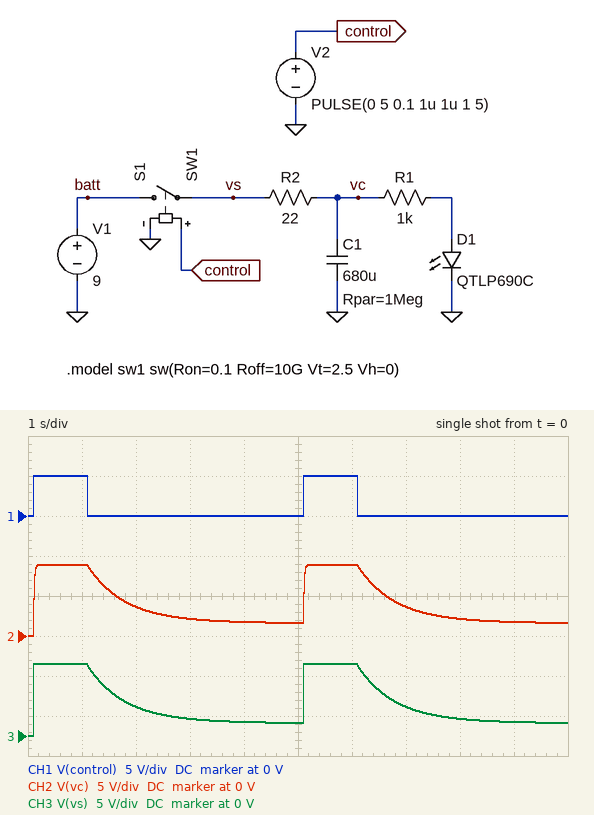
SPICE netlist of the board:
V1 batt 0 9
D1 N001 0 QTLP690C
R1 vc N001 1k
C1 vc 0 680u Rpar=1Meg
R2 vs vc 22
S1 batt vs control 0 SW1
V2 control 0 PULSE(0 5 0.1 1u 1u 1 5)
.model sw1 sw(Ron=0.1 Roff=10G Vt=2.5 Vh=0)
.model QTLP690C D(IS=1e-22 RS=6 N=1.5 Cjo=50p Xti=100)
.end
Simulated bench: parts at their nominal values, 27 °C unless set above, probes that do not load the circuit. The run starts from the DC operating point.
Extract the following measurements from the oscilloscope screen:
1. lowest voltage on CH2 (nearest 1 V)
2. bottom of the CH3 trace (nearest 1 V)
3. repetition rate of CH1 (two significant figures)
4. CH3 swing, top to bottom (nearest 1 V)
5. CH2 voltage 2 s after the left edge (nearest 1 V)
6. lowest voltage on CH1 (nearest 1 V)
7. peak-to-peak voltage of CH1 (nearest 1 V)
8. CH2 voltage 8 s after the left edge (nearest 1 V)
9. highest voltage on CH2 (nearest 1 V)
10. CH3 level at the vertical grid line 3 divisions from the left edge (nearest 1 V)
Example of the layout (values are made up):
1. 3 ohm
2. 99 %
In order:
1. 0 V
2. 0 V
3. 200 mHz
4. 9 V
5. 4 V
6. 0 V
7. 5 V
8. 2 V
9. 9 V
10. 2 V
